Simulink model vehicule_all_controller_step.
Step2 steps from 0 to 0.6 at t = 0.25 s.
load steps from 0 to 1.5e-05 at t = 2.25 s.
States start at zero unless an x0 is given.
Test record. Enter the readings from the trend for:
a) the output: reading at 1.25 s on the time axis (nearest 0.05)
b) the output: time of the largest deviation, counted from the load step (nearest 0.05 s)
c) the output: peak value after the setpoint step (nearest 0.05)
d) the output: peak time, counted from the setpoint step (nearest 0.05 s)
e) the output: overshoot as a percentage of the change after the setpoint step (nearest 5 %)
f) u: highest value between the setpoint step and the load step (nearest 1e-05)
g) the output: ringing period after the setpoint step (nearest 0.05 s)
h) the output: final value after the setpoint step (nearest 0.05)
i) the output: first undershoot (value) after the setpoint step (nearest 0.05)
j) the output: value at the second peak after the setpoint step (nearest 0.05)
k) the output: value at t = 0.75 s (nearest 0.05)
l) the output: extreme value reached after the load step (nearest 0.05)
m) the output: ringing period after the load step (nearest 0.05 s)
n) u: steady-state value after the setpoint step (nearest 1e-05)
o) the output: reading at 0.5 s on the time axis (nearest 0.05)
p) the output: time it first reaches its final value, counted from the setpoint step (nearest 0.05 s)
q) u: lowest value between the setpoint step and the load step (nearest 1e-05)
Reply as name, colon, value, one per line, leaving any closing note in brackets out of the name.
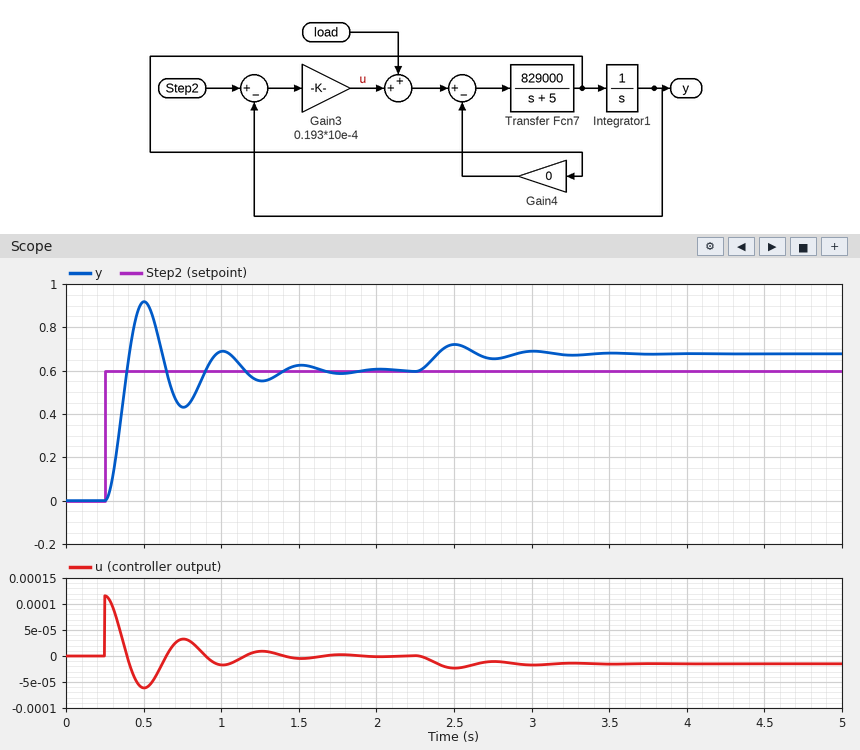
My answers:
the output: reading at 1.25 s on the time axis: 0.55
the output: time of the largest deviation, counted from the load step: 0.25 s
the output: peak value after the setpoint step: 0.90
the output: peak time, counted from the setpoint step: 0.25 s
the output: overshoot as a percentage of the change after the setpoint step: 55 %
u: highest value between the setpoint step and the load step: 0.00012
the output: ringing period after the setpoint step: 0.50 s
the output: final value after the setpoint step: 0.60
the output: first undershoot (value) after the setpoint step: 0.45
the output: value at the second peak after the setpoint step: 0.70
the output: value at t = 0.75 s: 0.45
the output: extreme value reached after the load step: 0.70
the output: ringing period after the load step: 0.50 s
u: steady-state value after the setpoint step: 0.00000
the output: reading at 0.5 s on the time axis: 0.90
the output: time it first reaches its final value, counted from the setpoint step: 0.15 s
u: lowest value between the setpoint step and the load step: -0.00006
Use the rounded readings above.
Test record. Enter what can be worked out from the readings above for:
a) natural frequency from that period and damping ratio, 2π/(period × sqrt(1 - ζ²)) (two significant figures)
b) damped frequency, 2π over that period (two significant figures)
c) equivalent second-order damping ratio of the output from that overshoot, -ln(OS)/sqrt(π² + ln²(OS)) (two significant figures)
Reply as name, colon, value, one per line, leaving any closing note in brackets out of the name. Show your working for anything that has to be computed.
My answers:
natural frequency from that period and damping ratio, 2π/(period × sqrt(1 - ζ²)): 2π / (0.5 × sqrt(1 - 0.19²)) = 13 rad/s
damped frequency, 2π over that period: 2π / 0.5 = 13 rad/s
equivalent second-order damping ratio of the output from that overshoot, -ln(OS)/sqrt(π² + ln²(OS)): ln(0.55) = -0.598; 0.598 / sqrt(9.870 + 0.357) = 0.19
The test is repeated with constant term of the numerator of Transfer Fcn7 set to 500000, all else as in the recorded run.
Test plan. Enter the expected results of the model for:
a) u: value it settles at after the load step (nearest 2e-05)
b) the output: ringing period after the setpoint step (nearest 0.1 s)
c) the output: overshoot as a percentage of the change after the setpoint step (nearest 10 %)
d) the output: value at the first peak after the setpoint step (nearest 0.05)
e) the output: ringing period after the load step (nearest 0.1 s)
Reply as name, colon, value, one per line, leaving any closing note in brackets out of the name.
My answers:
u: value it settles at after the load step: -0.00002
the output: ringing period after the setpoint step: 0.7 s
the output: overshoot as a percentage of the change after the setpoint step: 40 %
the output: value at the first peak after the setpoint step: 0.85
the output: ringing period after the load step: 0.7 s
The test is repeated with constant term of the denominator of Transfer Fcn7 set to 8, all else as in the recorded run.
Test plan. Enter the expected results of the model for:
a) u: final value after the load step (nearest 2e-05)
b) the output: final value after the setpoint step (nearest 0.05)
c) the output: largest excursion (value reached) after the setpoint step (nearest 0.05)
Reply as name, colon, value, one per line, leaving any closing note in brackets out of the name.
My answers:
u: final value after the load step: -0.00002
the output: final value after the setpoint step: 0.60
the output: largest excursion (value reached) after the setpoint step: 0.80
